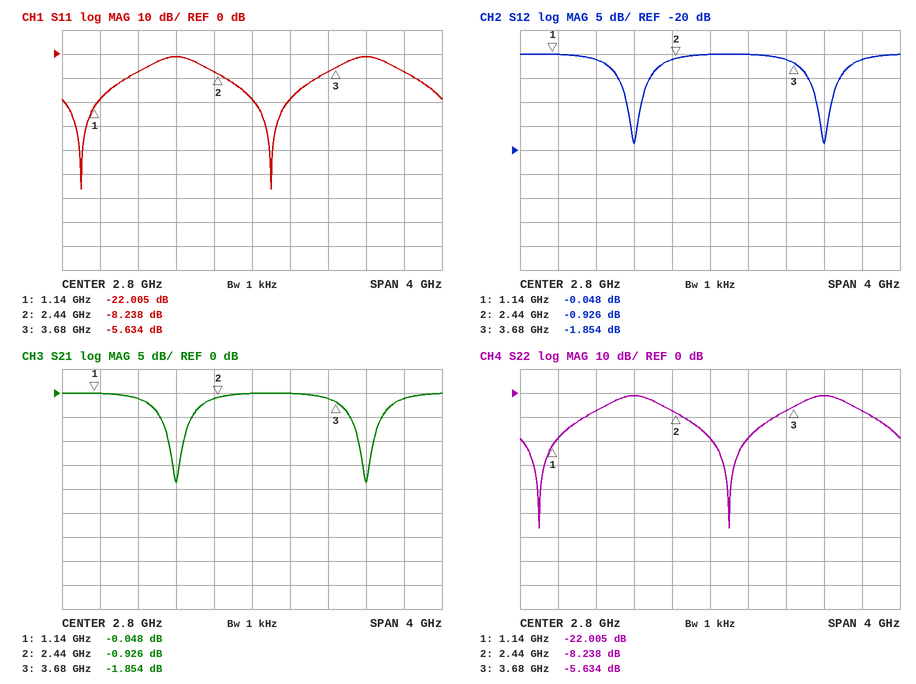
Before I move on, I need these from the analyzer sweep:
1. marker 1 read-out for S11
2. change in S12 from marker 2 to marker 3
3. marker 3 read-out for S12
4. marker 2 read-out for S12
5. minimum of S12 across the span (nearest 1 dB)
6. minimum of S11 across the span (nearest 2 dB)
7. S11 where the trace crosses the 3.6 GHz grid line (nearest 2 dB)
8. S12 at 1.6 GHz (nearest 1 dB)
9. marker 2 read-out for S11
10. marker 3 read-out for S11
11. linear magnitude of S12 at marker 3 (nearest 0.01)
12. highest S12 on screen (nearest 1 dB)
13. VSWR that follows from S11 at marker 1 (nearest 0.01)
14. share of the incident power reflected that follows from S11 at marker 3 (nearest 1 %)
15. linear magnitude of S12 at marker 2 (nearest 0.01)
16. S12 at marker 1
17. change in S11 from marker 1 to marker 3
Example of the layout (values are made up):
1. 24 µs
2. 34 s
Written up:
1. -22.005 dB
2. -0.928 dB
3. -1.854 dB
4. -0.926 dB
5. -19 dB
6. -56 dB
7. -8 dB
8. -1 dB
9. -8.238 dB
10. -5.634 dB
11. 0.81
12. 0 dB
13. 1.17
14. 27 %
15. 0.90
16. -0.048 dB
17. 16.371 dB
